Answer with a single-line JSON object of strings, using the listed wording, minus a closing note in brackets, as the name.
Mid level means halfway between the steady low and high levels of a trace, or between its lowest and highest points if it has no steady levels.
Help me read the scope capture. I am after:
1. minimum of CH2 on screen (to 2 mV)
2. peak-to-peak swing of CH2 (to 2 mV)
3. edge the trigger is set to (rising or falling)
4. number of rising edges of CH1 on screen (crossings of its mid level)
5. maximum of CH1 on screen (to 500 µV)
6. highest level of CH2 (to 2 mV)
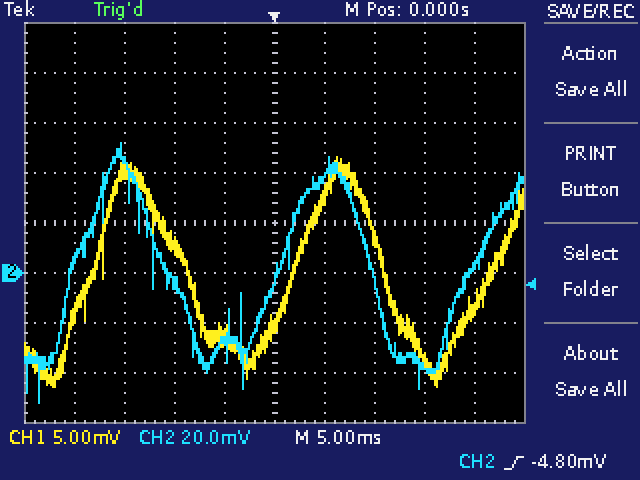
{"minimum of CH2 on screen": "-52 mV", "peak-to-peak swing of CH2": "104 mV", "edge the trigger is set to": "rising", "number of rising edges of CH1 on screen": "3", "maximum of CH1 on screen": "11.5 mV", "highest level of CH2": "52 mV"}
